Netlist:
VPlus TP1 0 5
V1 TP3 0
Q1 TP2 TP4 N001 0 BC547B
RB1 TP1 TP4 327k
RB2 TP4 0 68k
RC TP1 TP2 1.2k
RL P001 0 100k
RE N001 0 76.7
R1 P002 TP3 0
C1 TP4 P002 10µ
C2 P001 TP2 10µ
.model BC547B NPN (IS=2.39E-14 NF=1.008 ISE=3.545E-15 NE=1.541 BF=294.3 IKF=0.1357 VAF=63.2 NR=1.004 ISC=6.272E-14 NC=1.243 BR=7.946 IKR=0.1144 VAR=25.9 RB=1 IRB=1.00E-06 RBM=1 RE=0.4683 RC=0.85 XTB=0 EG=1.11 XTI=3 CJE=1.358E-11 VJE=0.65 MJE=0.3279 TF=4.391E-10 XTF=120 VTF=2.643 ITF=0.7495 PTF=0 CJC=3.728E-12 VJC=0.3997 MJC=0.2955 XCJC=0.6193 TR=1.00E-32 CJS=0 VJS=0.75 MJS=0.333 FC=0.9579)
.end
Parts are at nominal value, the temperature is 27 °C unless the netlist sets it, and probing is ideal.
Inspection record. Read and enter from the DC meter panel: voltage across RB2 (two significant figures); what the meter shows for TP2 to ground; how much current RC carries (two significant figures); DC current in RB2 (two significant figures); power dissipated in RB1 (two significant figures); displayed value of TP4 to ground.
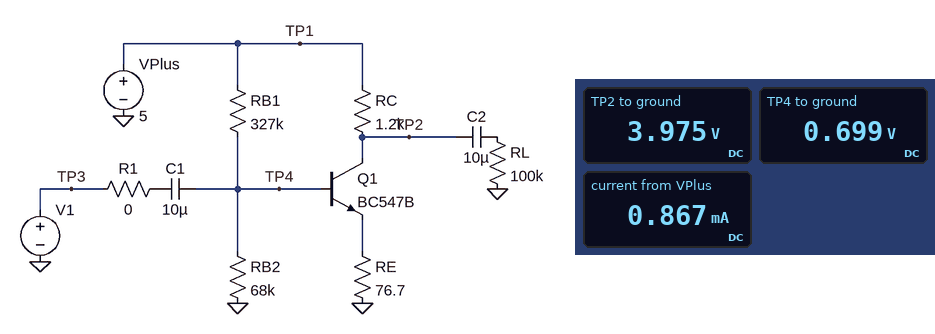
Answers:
700 mV
3.975 V
850 µA
10 µA
57 µW
0.699 V
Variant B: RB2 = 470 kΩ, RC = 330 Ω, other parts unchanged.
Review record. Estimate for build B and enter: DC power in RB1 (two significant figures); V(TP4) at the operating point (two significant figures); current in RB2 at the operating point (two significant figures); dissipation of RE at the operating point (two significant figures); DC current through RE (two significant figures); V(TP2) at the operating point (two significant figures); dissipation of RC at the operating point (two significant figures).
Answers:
51 µW
910 mV
1.9 µA
740 µW
3.1 mA
4.0 V
3.2 mW
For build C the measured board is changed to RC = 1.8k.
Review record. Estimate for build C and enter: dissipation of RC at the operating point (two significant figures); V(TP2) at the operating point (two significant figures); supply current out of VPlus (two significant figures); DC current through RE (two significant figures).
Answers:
1.3 mW
3.5 V
860 µA
850 µA
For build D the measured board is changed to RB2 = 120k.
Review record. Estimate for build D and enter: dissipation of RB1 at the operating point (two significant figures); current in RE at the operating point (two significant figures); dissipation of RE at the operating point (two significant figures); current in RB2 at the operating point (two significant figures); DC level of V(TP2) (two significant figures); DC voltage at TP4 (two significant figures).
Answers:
54 µW
1.8 mA
250 µW
6.6 µA
2.8 V
790 mV
